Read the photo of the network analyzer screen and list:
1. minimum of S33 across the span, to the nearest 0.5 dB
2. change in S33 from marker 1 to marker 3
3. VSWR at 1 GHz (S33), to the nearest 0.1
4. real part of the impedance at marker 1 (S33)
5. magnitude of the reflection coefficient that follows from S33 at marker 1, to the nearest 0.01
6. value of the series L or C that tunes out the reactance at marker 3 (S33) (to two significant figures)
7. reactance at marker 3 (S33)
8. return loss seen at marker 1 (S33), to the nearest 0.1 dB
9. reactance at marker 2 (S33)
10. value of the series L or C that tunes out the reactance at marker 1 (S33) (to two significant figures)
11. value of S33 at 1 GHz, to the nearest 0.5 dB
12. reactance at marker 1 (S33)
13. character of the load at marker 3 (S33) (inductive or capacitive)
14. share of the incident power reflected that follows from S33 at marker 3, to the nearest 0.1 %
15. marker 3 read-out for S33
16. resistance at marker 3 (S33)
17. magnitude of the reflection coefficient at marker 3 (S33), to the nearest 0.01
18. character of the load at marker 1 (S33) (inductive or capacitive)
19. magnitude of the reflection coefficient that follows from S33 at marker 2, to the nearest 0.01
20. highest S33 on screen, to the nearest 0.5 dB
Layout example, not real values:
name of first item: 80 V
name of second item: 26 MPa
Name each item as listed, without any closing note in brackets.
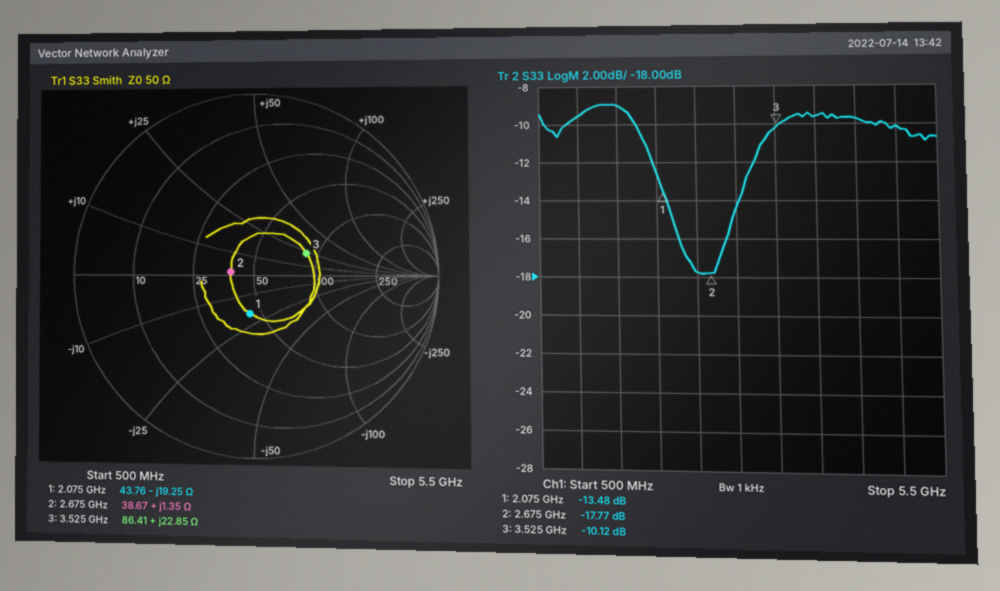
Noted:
minimum of S33 across the span, to the nearest 0.5 dB: -18.0 dB
change in S33 from marker 1 to marker 3: 3.36 dB
VSWR at 1 GHz (S33), to the nearest 0.1: 2.0
real part of the impedance at marker 1: 43.76 Ω
magnitude of the reflection coefficient that follows from S33 at marker 1, to the nearest 0.01: 0.21
value of the series L or C that tunes out the reactance at marker 3 (S33): 2.0 pF
reactance at marker 3: +22.85 Ω
return loss seen at marker 1 (S33), to the nearest 0.1 dB: 13.5 dB
reactance at marker 2: +1.35 Ω
value of the series L or C that tunes out the reactance at marker 1 (S33): 1.5 nH
value of S33 at 1 GHz, to the nearest 0.5 dB: -9.5 dB
reactance at marker 1: -19.25 Ω
character of the load at marker 3 (S33): inductive
share of the incident power reflected that follows from S33 at marker 3, to the nearest 0.1 %: 9.7 %
marker 3 read-out for S33: -10.12 dB
resistance at marker 3: 86.41 Ω
magnitude of the reflection coefficient at marker 3 (S33), to the nearest 0.01: 0.31
character of the load at marker 1 (S33): capacitive
magnitude of the reflection coefficient that follows from S33 at marker 2, to the nearest 0.01: 0.13
highest S33 on screen, to the nearest 0.5 dB: -9.0 dB
